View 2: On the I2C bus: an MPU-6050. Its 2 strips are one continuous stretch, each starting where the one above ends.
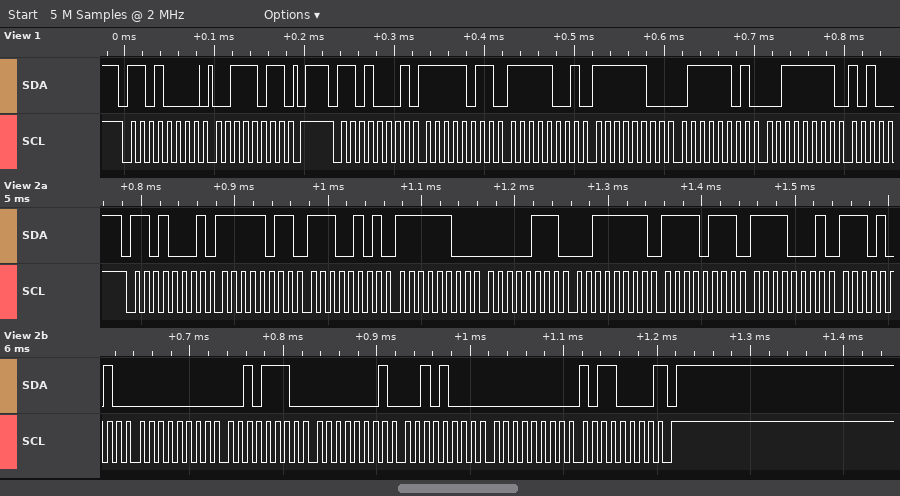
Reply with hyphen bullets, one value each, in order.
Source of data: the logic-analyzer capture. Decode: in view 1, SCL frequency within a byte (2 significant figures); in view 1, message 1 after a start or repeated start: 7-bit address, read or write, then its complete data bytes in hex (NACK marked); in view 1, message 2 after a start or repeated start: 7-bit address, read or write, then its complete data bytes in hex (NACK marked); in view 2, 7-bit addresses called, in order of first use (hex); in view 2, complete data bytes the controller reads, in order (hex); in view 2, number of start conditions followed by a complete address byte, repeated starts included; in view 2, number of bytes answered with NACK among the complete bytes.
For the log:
- 100 kHz
- 0x68 write: 3B
- 0x68 read: FB F9 FC 7D 3F
- 0x68
- FB E5 FC 07 3F F7 F1 EA 00 2E 01 28 00 B0
- 1
- 1
